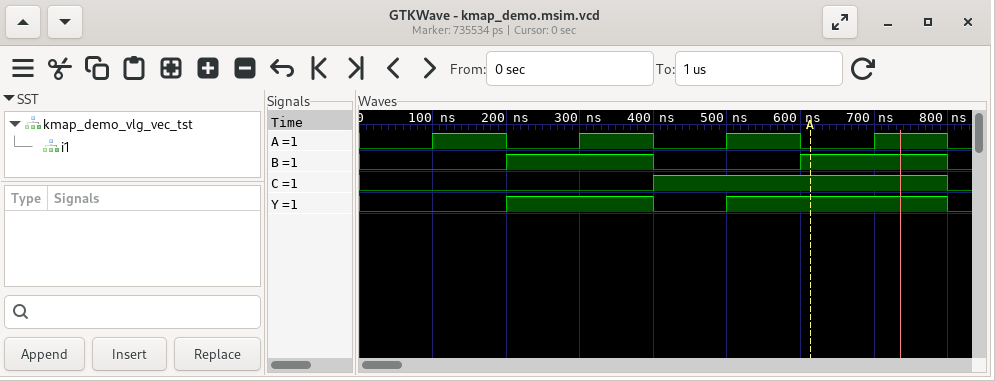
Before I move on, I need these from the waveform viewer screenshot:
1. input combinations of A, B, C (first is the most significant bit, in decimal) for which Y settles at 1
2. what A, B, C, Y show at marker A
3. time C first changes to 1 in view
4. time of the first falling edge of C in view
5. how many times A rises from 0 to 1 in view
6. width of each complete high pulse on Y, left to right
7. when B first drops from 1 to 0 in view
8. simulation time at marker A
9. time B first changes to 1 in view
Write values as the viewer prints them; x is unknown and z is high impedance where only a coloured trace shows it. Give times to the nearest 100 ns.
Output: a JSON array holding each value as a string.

["2, 3, 5, 6, 7", "A=0, B=1, C=1, Y=1", "400 ns", "800 ns", "4", "200 ns, 300 ns", "400 ns", "600 ns", "200 ns"]
